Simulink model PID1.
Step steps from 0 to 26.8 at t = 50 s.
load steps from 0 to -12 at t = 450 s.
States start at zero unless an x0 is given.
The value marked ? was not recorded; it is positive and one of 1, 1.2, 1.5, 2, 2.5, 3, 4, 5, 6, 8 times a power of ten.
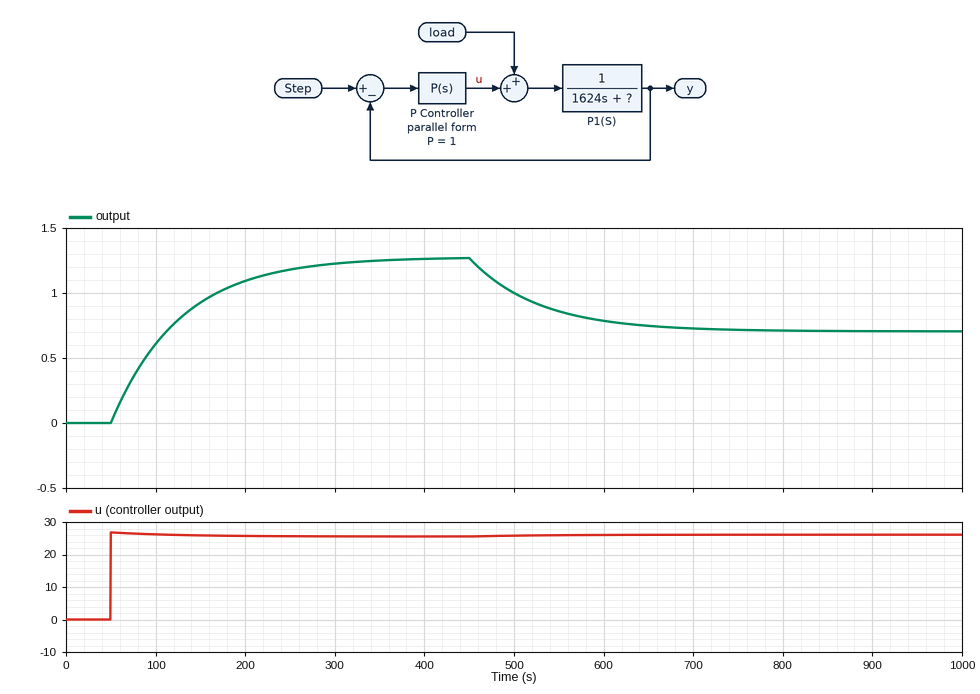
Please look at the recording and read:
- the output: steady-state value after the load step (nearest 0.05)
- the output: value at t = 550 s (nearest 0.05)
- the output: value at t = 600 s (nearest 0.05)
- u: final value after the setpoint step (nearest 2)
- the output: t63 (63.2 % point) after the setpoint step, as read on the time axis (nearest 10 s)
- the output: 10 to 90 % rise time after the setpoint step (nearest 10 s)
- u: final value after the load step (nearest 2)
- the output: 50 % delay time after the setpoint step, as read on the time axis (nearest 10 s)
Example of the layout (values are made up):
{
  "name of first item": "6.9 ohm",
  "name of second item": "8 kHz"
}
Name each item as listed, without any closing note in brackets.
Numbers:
{
  "the output: steady-state value after the load step": "0.70",
  "the output: value at t = 550 s": "0.85",
  "the output: value at t = 600 s": "0.80",
  "u: final value after the setpoint step": "26",
  "the output: t63 (63.2 % point) after the setpoint step, as read on the time axis": "130 s",
  "the output: 10 to 90 % rise time after the setpoint step": "170 s",
  "u: final value after the load step": "26",
  "the output: 50 % delay time after the setpoint step, as read on the time axis": "100 s"
}
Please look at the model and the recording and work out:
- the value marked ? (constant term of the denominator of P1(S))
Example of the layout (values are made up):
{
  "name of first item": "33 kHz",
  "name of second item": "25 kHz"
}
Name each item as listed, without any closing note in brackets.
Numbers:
{
  "the value marked ? (constant term of the denominator of P1(S))": "20"
}
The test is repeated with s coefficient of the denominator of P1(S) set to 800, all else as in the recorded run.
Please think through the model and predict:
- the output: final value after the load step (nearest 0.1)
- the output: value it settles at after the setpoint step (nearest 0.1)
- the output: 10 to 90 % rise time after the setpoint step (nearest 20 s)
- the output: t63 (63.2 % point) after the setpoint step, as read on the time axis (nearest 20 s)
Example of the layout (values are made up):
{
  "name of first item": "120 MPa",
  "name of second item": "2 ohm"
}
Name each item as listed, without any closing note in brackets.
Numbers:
{
  "the output: final value after the load step": "0.7",
  "the output: value it settles at after the setpoint step": "1.3",
  "the output: 10 to 90 % rise time after the setpoint step": "80 s",
  "the output: t63 (63.2 % point) after the setpoint step, as read on the time axis": "80 s"
}
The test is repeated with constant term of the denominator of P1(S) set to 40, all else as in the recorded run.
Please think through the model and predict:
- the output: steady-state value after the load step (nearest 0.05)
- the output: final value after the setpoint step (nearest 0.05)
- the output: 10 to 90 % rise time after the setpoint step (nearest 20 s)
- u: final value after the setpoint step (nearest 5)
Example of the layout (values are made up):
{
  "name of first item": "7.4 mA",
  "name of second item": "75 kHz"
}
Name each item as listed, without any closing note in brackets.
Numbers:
{
  "the output: steady-state value after the load step": "0.35",
  "the output: final value after the setpoint step": "0.65",
  "the output: 10 to 90 % rise time after the setpoint step": "80 s",
  "u: final value after the setpoint step": "25"
}
